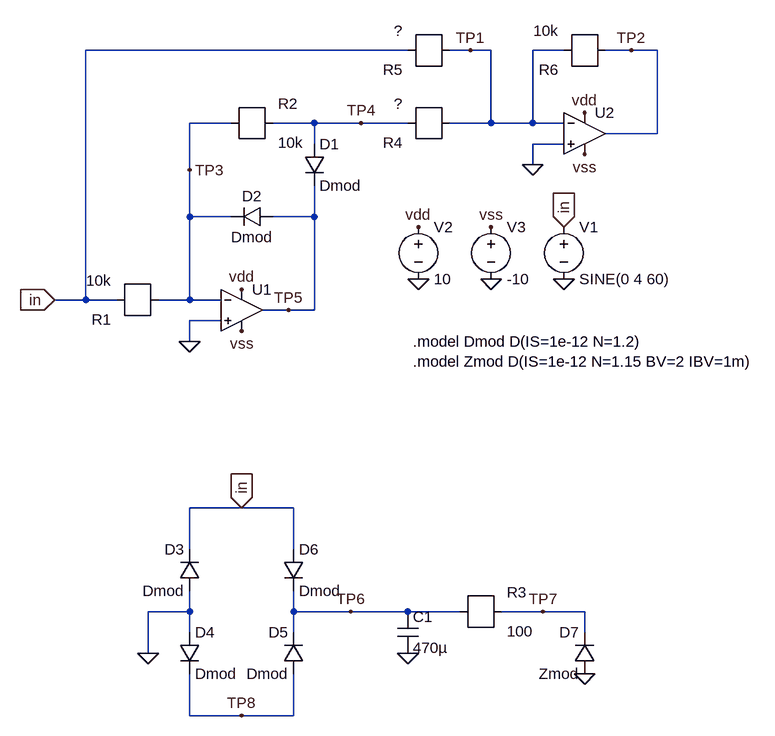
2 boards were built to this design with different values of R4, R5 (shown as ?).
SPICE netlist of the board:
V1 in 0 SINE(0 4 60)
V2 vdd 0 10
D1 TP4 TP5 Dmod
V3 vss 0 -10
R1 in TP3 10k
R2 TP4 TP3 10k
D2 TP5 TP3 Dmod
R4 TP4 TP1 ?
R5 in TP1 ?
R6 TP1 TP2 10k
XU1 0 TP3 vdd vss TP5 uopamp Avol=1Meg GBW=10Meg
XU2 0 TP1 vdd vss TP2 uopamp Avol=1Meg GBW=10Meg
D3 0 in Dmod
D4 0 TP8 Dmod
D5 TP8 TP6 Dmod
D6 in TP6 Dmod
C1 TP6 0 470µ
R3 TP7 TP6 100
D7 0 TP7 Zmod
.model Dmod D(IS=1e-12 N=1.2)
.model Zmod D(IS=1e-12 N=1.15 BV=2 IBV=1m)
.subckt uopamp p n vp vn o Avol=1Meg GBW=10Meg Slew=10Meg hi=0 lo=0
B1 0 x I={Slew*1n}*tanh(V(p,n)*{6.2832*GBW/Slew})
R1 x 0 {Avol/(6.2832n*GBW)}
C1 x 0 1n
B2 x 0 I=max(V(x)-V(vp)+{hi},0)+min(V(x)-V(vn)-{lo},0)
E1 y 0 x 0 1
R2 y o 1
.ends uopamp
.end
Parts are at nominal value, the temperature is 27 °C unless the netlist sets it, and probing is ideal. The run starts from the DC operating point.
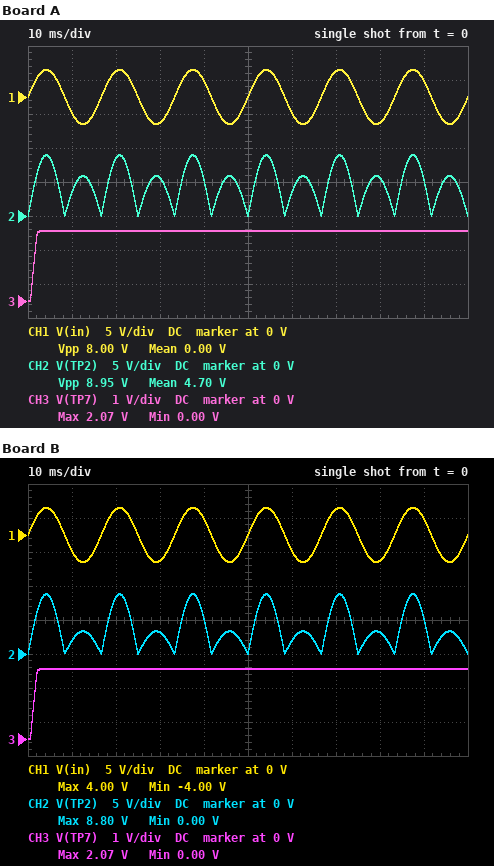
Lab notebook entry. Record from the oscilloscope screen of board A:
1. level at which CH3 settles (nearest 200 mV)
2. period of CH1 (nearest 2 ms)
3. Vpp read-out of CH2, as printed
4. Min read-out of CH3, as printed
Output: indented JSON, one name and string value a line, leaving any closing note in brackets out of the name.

{
  "level at which CH3 settles": "2.0 V",
  "period of CH1": "16 ms",
  "Vpp read-out of CH2, as printed": "8.95 V",
  "Min read-out of CH3, as printed": "0.00 V"
}
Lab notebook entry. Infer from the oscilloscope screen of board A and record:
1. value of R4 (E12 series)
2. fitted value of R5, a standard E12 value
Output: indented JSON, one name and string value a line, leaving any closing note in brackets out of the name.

{
  "value of R4": "2.7 kΩ",
  "fitted value of R5, a standard E12 value": "6.8 kΩ"
}
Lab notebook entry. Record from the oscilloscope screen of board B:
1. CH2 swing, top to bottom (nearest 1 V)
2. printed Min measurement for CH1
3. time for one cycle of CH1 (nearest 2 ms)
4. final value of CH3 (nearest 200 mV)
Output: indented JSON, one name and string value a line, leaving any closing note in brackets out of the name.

{
  "CH2 swing, top to bottom": "9 V",
  "printed Min measurement for CH1": "-4.00 V",
  "time for one cycle of CH1": "16 ms",
  "final value of CH3": "2.0 V"
}
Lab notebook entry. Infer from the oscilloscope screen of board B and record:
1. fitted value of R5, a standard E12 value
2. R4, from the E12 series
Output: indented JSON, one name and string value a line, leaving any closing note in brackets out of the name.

{
  "fitted value of R5, a standard E12 value": "12 kΩ",
  "R4, from the E12 series": "3.3 kΩ"
}
